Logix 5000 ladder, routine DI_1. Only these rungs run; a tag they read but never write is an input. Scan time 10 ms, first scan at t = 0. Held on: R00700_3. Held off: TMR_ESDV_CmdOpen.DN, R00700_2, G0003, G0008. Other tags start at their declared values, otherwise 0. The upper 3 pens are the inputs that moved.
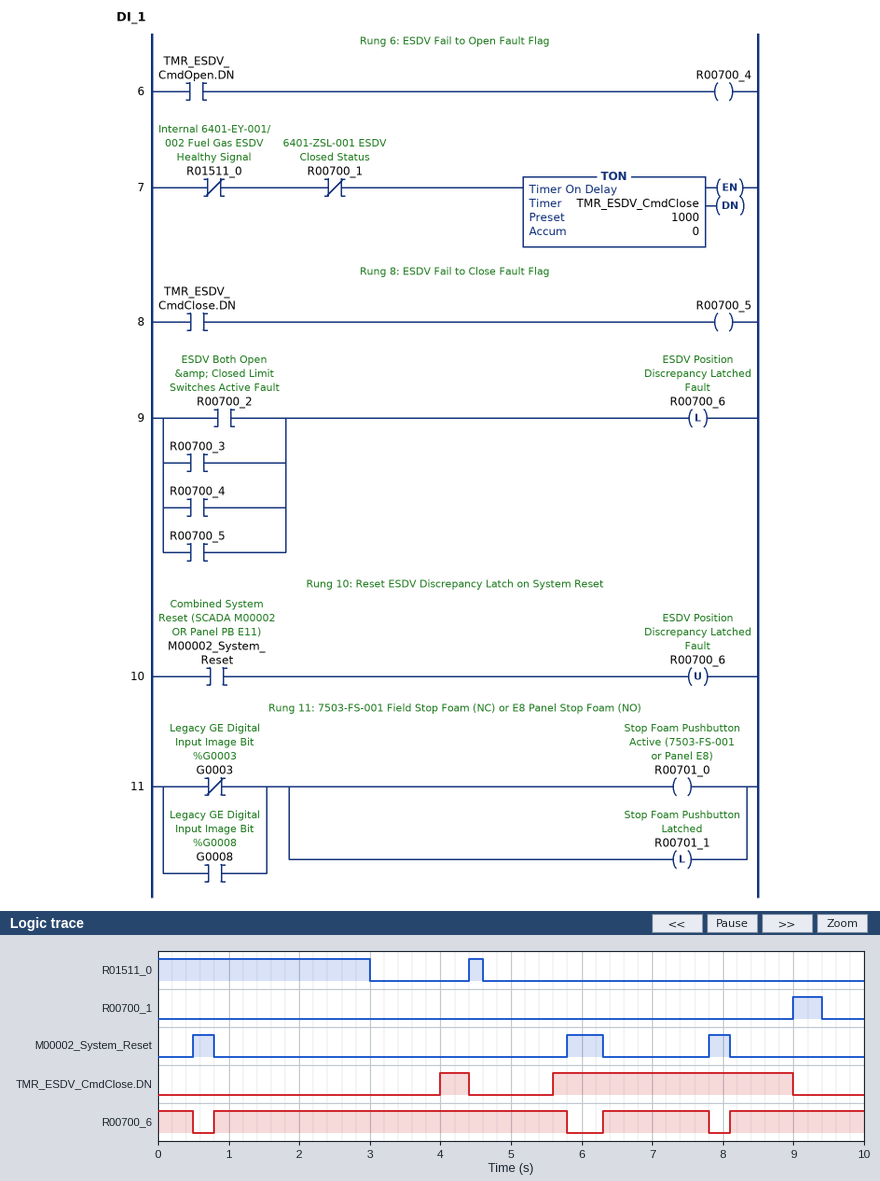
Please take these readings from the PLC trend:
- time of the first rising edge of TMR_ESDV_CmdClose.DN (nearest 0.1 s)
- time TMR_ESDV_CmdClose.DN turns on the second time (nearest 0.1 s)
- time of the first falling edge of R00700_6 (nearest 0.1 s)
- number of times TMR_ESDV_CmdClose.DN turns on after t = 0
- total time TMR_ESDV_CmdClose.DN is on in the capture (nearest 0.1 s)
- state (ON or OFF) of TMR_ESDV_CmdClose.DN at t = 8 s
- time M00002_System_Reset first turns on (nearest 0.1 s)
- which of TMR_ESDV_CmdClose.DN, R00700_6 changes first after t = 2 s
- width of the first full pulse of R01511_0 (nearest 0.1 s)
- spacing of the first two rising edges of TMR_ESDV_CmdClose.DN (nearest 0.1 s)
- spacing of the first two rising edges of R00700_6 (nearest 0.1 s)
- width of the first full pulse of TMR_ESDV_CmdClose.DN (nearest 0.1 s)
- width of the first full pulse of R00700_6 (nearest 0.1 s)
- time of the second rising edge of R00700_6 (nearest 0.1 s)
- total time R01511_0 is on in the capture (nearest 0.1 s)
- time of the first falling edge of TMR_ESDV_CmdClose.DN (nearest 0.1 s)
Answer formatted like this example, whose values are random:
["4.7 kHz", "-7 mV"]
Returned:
["4.0 s", "5.6 s", "0.5 s", "2", "3.8 s", "ON", "0.5 s", "TMR_ESDV_CmdClose.DN", "0.2 s", "1.6 s", "5.5 s", "0.4 s", "5.0 s", "6.3 s", "3.2 s", "4.4 s"]
